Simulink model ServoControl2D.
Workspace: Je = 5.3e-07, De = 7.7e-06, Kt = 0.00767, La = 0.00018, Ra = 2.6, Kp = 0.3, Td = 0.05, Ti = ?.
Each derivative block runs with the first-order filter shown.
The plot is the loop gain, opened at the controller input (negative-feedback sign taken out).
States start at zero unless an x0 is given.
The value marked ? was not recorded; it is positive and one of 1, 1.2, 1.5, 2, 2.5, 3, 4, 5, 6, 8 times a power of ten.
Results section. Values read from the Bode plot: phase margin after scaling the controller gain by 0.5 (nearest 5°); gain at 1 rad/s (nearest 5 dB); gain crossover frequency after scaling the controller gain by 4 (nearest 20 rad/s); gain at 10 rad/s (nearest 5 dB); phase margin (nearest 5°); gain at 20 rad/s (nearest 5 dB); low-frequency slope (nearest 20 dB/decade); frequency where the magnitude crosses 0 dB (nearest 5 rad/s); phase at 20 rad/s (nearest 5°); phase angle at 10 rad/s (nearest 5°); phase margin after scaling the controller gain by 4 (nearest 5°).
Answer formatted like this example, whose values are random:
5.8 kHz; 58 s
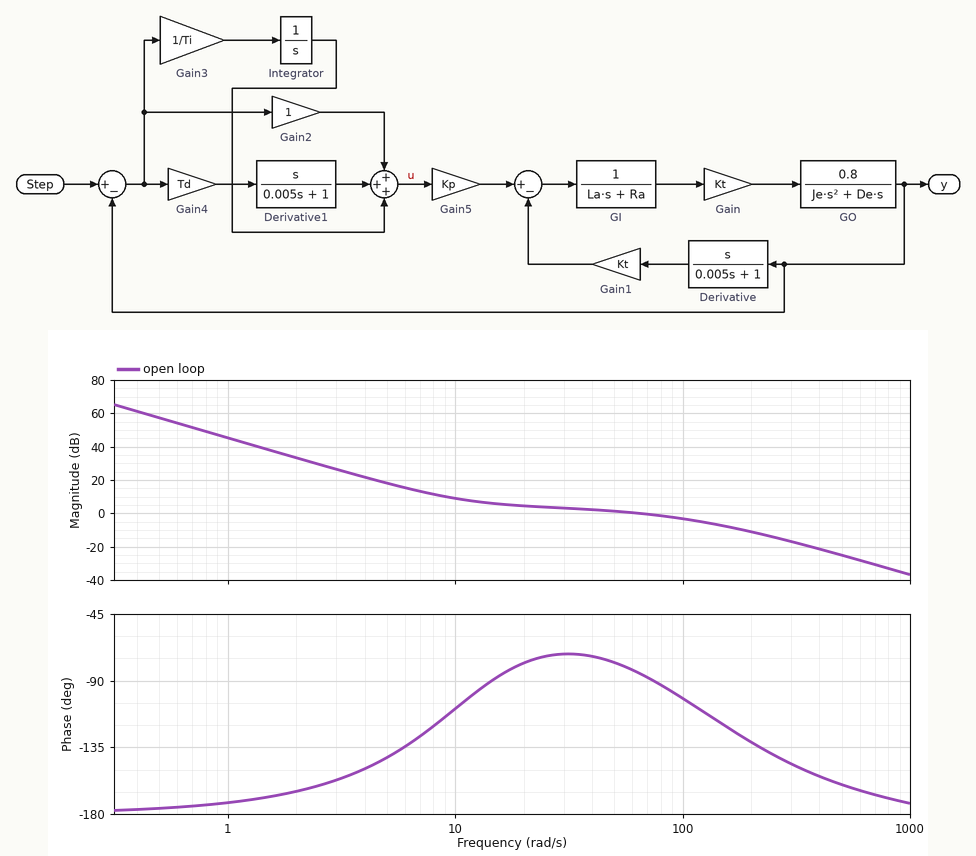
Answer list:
90°; 45 dB; 220 rad/s; 10 dB; 95°; 5 dB; -40 dB/decade; 65 rad/s; -80°; -110°; 45°
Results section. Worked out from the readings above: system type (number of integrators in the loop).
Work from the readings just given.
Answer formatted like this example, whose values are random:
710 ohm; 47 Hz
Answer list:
2
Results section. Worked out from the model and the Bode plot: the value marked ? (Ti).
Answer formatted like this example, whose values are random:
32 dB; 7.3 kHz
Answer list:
0.15
